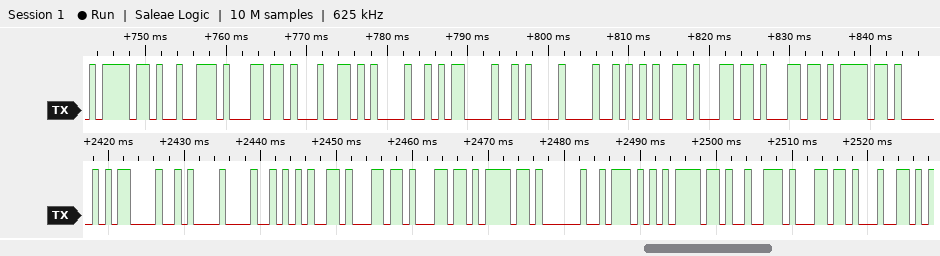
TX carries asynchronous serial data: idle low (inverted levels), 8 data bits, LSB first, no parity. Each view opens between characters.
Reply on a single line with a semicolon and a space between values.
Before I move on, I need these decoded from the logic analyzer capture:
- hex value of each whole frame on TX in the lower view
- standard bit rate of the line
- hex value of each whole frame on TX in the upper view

E5, EB, 6F, 35, 27, 27, 21, BF, 51, 21, 1B, 27, 37; 1200 baud; 21, 1B, 27, 37, BD, E5, EB, 6F, 35, 27, 27, 21
